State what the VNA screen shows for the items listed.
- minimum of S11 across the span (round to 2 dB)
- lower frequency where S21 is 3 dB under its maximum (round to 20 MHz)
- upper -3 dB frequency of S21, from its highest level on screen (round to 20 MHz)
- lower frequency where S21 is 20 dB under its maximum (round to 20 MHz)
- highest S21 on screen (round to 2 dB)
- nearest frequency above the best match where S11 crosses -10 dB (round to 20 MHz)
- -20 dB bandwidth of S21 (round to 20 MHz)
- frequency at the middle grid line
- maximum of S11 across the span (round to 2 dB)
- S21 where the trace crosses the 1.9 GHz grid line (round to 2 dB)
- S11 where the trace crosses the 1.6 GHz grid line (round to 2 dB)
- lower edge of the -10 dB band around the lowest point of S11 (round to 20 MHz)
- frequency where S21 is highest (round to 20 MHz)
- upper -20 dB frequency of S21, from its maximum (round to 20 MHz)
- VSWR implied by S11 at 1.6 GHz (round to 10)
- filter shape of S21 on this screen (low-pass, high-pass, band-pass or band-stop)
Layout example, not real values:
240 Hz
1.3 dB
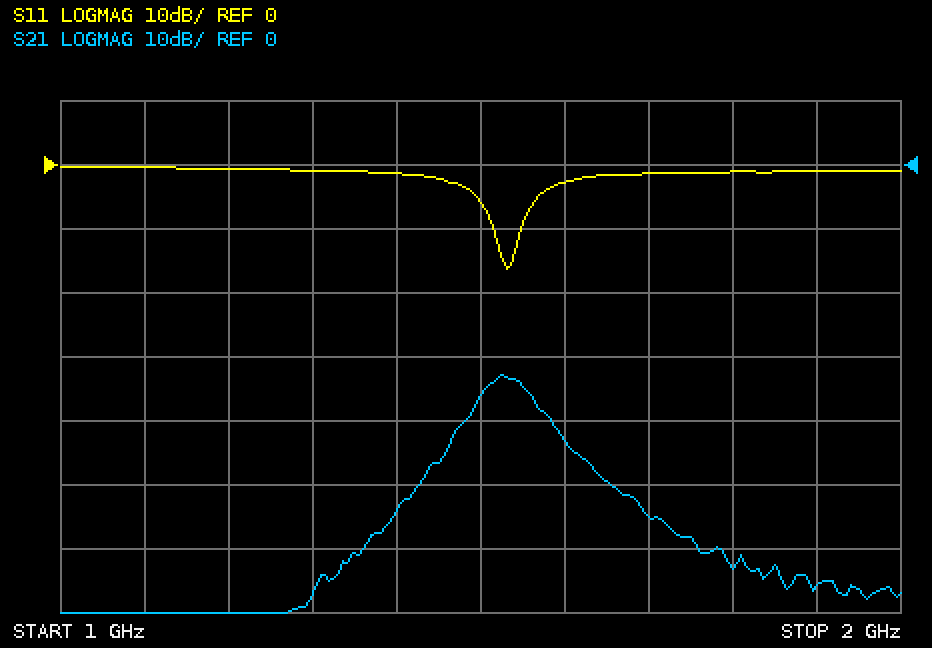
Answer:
-16 dB
1.50 GHz
1.56 GHz
1.40 GHz
-32 dB
1.54 GHz
280 MHz
1.5 GHz
0 dB
-66 dB
-2 dB
1.52 GHz
1.52 GHz
1.68 GHz
10
band-pass
